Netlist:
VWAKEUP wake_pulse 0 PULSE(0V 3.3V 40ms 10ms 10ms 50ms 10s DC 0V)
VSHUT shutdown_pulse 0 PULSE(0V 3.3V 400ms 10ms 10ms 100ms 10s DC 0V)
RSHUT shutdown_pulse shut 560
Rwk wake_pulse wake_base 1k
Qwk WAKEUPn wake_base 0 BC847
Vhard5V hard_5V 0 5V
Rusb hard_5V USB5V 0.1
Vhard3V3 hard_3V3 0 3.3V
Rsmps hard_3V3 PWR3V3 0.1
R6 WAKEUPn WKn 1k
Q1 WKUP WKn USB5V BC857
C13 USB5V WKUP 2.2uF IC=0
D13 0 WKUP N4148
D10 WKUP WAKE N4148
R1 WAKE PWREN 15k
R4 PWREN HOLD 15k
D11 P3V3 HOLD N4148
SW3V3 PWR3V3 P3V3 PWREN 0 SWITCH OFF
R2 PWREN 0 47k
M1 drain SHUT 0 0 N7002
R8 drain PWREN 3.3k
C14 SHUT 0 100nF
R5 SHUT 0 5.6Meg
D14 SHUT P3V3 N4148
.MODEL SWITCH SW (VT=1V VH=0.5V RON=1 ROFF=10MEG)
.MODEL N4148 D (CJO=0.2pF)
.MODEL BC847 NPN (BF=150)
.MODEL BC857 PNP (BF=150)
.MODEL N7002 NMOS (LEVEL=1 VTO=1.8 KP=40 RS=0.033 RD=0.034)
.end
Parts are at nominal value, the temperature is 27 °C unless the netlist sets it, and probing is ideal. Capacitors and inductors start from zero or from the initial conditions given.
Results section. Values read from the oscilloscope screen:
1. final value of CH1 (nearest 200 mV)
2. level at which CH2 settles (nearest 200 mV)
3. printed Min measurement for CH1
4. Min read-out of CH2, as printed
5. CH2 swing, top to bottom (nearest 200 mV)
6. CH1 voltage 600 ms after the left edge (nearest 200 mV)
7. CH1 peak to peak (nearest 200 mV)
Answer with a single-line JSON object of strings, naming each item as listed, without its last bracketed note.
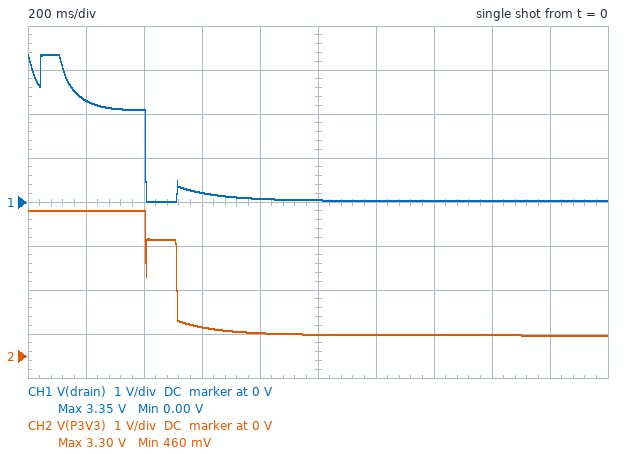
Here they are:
{"final value of CH1": "0 V", "level at which CH2 settles": "400 mV", "printed Min measurement for CH1": "0.00 V", "Min read-out of CH2, as printed": "460 mV", "CH2 swing, top to bottom": "2.8 V", "CH1 voltage 600 ms after the left edge": "200 mV", "CH1 peak to peak": "3.4 V"}
